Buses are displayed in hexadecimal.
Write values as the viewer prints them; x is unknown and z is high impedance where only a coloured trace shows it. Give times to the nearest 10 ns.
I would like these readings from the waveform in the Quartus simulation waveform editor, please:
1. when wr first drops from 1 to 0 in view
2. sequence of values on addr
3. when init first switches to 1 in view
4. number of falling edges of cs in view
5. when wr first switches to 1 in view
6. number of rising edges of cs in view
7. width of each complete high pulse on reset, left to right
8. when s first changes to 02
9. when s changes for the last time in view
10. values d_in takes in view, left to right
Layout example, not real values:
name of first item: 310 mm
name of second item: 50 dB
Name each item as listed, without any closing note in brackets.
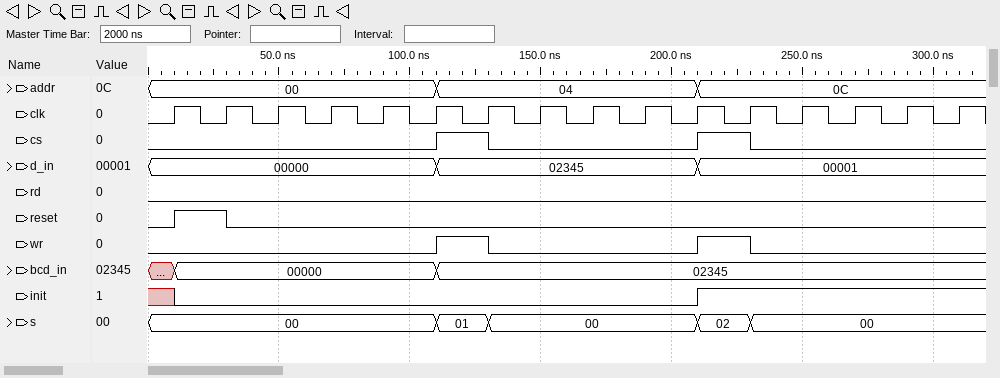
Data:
when wr first drops from 1 to 0 in view: 130 ns
sequence of values on addr: 00, 04, 0C
when init first switches to 1 in view: 210 ns
number of falling edges of cs in view: 2
when wr first switches to 1 in view: 110 ns
number of rising edges of cs in view: 2
width of each complete high pulse on reset, left to right: 20 ns
when s first changes to 02: 210 ns
when s changes for the last time in view: 230 ns
values d_in takes in view, left to right: 00000, 02345, 00001
